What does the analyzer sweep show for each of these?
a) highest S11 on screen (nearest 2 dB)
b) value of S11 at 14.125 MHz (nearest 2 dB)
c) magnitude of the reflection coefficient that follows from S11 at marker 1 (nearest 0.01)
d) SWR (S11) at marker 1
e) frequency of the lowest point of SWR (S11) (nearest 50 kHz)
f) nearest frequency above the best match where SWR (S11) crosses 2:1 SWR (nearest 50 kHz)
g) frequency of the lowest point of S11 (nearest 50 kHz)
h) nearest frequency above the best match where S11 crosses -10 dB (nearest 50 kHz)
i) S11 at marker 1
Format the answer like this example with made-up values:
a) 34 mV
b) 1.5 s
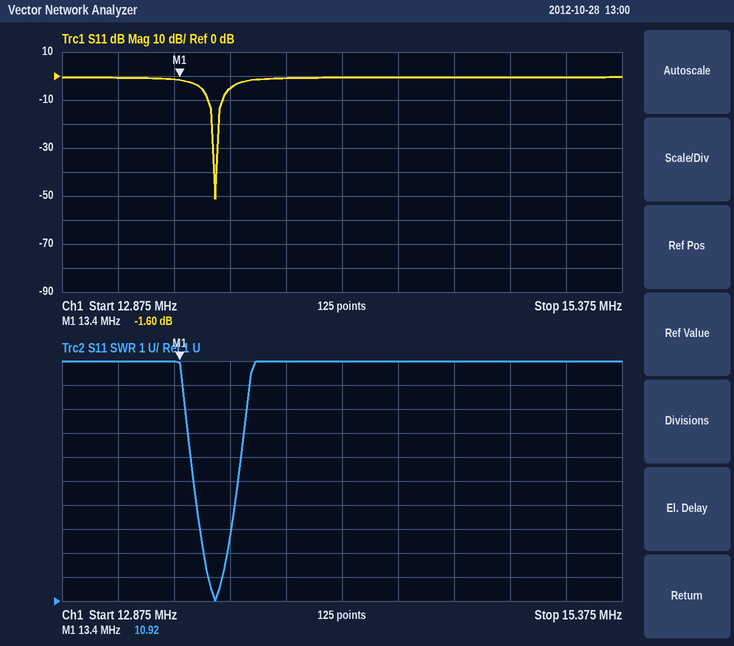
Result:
a) 0 dB
b) 0 dB
c) 0.83
d) 10.92
e) 13.55 MHz
f) 13.60 MHz
g) 13.55 MHz
h) 13.60 MHz
i) -1.60 dB
